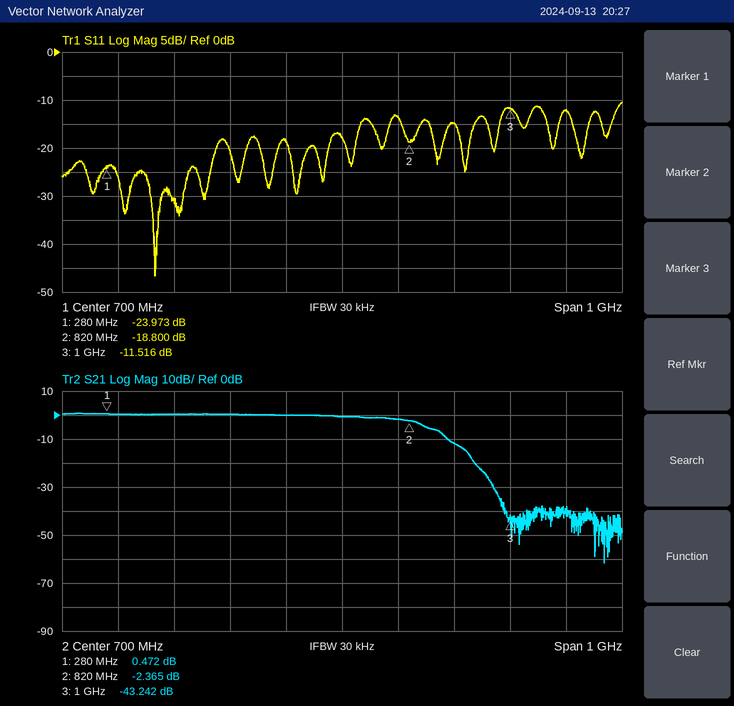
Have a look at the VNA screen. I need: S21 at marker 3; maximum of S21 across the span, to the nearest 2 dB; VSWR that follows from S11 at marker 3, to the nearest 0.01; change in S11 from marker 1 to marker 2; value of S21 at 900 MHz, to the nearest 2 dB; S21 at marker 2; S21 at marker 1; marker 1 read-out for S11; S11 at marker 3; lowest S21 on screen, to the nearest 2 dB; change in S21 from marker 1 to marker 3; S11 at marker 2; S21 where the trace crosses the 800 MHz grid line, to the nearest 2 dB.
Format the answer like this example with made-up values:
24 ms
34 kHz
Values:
-43.242 dB
0 dB
1.72
5.173 dB
-12 dB
-2.365 dB
0.472 dB
-23.973 dB
-11.516 dB
-62 dB
-43.714 dB
-18.800 dB
-2 dB
